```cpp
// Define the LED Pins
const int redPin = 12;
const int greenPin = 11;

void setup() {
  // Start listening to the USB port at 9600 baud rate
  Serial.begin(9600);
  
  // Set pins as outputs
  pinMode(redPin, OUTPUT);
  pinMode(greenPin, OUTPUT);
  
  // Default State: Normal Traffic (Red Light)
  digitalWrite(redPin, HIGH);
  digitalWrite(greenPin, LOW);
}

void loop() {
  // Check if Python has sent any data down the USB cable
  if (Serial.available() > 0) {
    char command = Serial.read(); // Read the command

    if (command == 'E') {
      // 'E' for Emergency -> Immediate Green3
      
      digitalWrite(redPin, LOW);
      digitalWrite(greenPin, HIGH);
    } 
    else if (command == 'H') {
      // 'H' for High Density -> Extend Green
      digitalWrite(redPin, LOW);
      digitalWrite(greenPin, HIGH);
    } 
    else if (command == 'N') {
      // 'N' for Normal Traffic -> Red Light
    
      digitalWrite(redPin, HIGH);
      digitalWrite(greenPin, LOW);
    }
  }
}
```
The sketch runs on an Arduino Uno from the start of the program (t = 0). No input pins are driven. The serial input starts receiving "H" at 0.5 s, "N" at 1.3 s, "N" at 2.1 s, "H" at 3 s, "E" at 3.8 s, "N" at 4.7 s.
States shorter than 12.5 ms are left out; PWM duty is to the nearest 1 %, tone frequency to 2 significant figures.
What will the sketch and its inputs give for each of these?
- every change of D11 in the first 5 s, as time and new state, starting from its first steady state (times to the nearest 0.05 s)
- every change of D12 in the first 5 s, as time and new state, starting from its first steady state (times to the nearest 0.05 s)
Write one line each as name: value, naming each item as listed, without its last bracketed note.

every change of D11 in the first 5 s, as time and new state, starting from its first steady state: 0 s low; 0.5 s high; 1.3 s low; 3 s high; 4.7 s low
every change of D12 in the first 5 s, as time and new state, starting from its first steady state: 0 s high; 0.5 s low; 1.3 s high; 3 s low; 4.7 s high
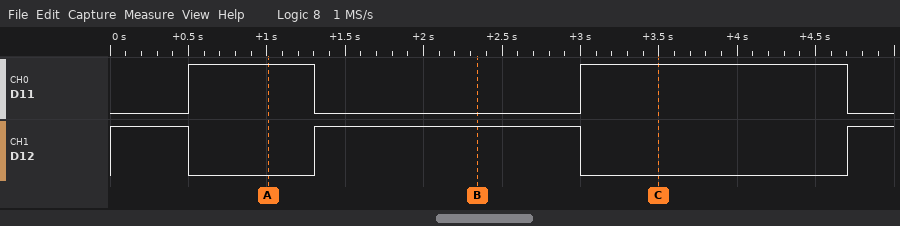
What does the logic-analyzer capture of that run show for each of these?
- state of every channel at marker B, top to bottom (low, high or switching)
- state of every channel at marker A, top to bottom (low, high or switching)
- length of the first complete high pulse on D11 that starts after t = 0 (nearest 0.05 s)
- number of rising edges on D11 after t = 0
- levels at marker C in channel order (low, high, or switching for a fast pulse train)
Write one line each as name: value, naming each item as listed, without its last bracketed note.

state of every channel at marker B, top to bottom: D11 low, D12 high
state of every channel at marker A, top to bottom: D11 high, D12 low
length of the first complete high pulse on D11 that starts after t = 0: 0.80 s
number of rising edges on D11 after t = 0: 2
levels at marker C in channel order: D11 high, D12 low
